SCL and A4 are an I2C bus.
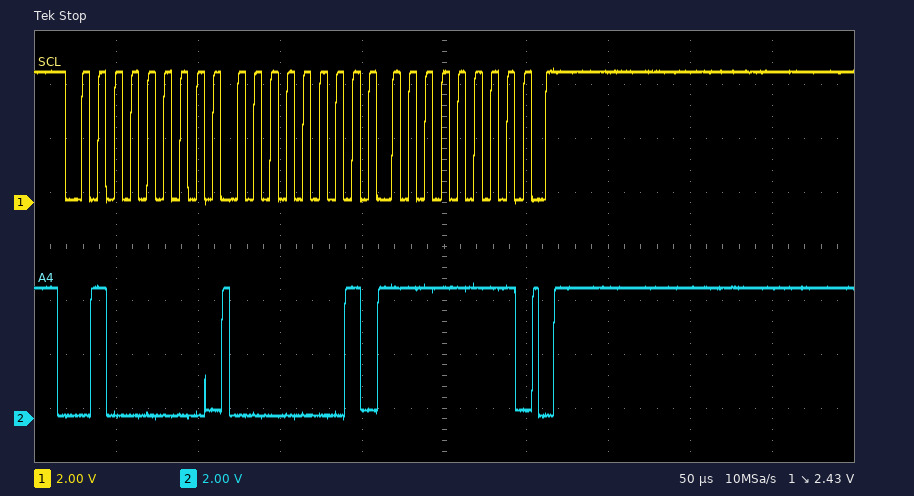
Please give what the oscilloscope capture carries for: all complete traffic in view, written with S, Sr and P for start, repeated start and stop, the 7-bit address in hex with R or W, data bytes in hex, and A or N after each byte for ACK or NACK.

S 20W A 01 A FF A P
